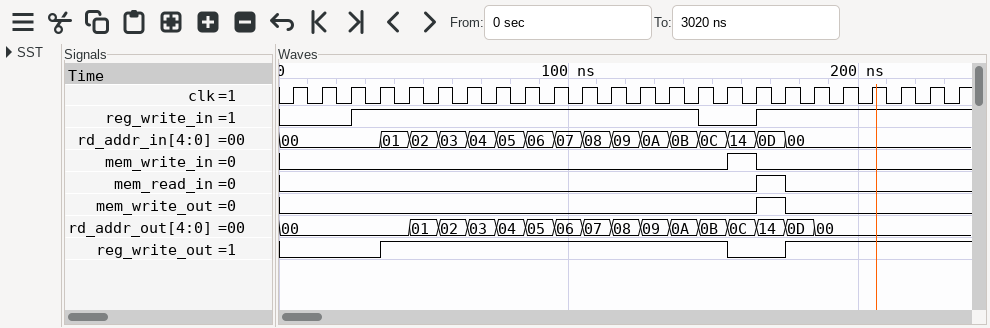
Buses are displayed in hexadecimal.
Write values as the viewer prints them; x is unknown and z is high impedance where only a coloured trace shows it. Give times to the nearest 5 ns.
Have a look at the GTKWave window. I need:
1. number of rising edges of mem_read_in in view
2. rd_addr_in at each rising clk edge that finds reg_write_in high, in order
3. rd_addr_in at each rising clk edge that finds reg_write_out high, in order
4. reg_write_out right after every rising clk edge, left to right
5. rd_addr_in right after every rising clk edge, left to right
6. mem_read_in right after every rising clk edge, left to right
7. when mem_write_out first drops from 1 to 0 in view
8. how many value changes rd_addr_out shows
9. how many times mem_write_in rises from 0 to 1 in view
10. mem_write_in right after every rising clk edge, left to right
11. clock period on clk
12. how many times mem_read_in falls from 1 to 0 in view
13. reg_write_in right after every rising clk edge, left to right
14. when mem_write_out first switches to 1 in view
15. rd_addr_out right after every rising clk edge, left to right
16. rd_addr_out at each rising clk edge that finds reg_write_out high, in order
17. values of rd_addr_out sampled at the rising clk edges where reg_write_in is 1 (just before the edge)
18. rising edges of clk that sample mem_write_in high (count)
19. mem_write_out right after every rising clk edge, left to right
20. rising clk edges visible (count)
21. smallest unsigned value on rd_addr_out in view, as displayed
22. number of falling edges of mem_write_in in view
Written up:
1
00, 01, 02, 03, 04, 05, 06, 07, 08, 09, 0A, 0B, 0D, 00, 00, 00, 00, 00, 00
01, 02, 03, 04, 05, 06, 07, 08, 09, 0A, 0B, 0C, 00, 00, 00, 00, 00, 00
0 0 0 1 1 1 1 1 1 1 1 1 1 1 1 0 0 1 1 1 1 1 1 1
00, 00, 00, 01, 02, 03, 04, 05, 06, 07, 08, 09, 0A, 0B, 0C, 14, 0D, 00, 00, 00, 00, 00, 00, 00
0 0 0 0 0 0 0 0 0 0 0 0 0 0 0 0 1 0 0 0 0 0 0 0
175 ns
15
1
0 0 0 0 0 0 0 0 0 0 0 0 0 0 0 1 0 0 0 0 0 0 0 0
10 ns
1
0 0 1 1 1 1 1 1 1 1 1 1 1 1 0 0 1 1 1 1 1 1 1 1
165 ns
00, 00, 00, 00, 01, 02, 03, 04, 05, 06, 07, 08, 09, 0A, 0B, 0C, 14, 0D, 00, 00, 00, 00, 00, 00
00, 01, 02, 03, 04, 05, 06, 07, 08, 09, 0A, 0B, 0D, 00, 00, 00, 00, 00
00, 00, 01, 02, 03, 04, 05, 06, 07, 08, 09, 0A, 14, 0D, 00, 00, 00, 00, 00
1
0 0 0 0 0 0 0 0 0 0 0 0 0 0 0 0 1 0 0 0 0 0 0 0
24
00
1
